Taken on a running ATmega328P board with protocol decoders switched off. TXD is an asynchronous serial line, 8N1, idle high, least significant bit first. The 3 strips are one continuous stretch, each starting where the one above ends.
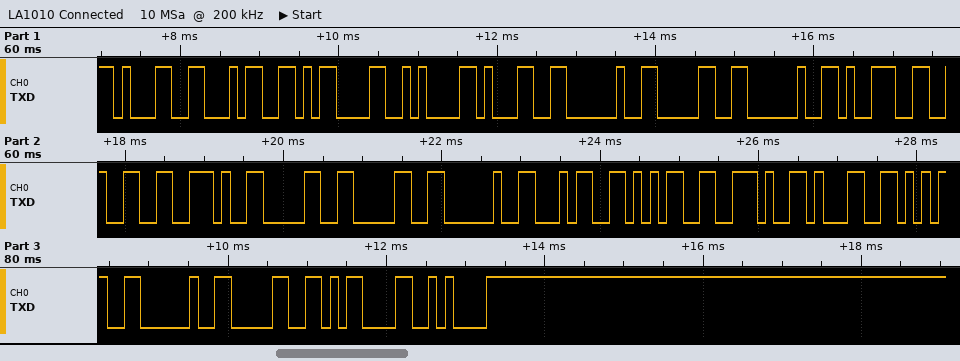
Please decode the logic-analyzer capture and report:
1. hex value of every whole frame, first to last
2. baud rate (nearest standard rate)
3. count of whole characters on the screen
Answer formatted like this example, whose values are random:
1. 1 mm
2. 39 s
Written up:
1. 31 34 0D 0A 31 20 30 20 39 32 2E 30 30 20 34 35 2E 31 35 20 30 0D 0A
2. 9600 baud
3. 23
